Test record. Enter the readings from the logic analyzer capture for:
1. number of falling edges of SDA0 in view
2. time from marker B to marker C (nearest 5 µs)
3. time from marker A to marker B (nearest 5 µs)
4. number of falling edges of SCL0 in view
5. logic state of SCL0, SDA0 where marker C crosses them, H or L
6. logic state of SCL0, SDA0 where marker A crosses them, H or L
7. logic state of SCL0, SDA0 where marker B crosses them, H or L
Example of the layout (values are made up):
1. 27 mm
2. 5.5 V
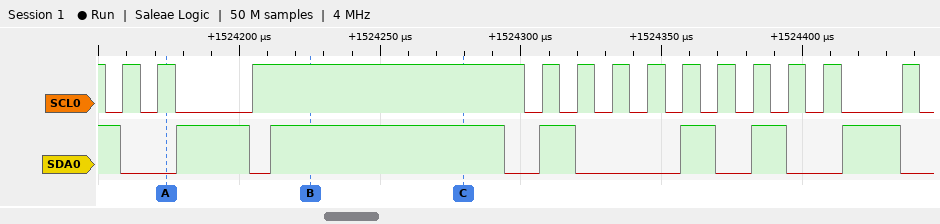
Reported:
1. 7
2. 55 µs
3. 50 µs
4. 14
5. SCL0=H, SDA0=H
6. SCL0=H, SDA0=L
7. SCL0=H, SDA0=H
